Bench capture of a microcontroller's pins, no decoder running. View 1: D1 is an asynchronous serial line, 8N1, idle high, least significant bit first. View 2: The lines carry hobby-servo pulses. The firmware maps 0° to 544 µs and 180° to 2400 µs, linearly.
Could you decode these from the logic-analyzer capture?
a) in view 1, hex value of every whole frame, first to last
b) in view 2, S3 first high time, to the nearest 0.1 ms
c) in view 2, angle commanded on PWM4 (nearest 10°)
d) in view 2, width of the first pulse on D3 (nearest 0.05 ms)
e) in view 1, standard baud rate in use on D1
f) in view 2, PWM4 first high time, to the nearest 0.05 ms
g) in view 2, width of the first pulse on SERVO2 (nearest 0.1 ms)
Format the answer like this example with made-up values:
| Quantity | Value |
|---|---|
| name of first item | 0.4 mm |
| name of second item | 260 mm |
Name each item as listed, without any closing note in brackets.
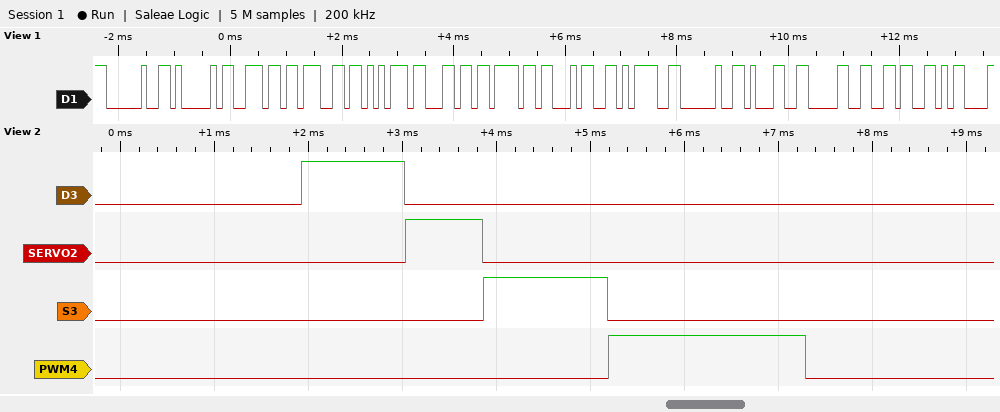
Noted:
| Quantity | Value |
|---|---|
| in view 1, hex value of every whole frame, first to last | 20 41 6E 67 75 6C 6F 34 3D 20 31 30 36 0D |
| in view 2, S3 first high time, to the nearest 0.1 ms | 1.3 ms |
| in view 2, angle commanded on PWM4 | 150° |
| in view 2, width of the first pulse on D3 | 1.10 ms |
| in view 1, standard baud rate in use on D1 | 9600 baud |
| in view 2, PWM4 first high time, to the nearest 0.05 ms | 2.10 ms |
| in view 2, width of the first pulse on SERVO2 | 0.8 ms |
